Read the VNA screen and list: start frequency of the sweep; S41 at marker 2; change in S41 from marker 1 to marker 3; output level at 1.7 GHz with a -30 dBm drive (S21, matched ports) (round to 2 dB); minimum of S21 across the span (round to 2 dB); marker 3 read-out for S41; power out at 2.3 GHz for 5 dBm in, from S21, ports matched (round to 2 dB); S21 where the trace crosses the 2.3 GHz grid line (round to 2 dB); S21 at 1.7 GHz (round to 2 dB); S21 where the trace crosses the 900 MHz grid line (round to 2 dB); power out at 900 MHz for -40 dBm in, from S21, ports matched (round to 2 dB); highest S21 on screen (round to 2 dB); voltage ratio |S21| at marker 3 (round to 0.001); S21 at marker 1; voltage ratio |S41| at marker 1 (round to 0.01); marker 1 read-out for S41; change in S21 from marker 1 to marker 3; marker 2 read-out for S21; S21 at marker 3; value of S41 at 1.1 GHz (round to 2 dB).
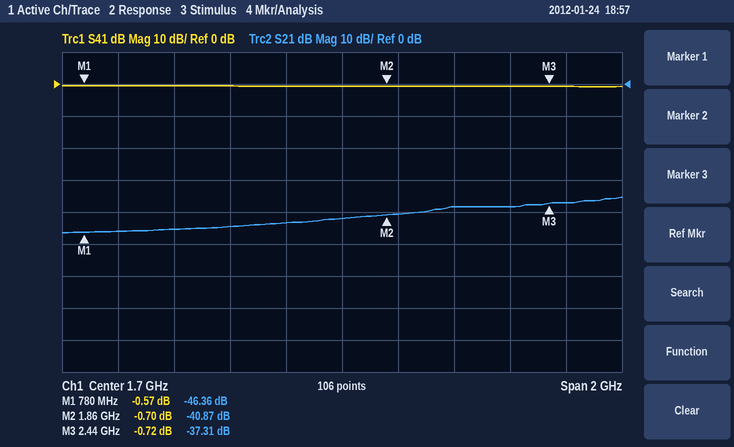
700 MHz
-0.70 dB
-0.15 dB
-72 dBm
-46 dB
-0.72 dB
-34 dBm
-38 dB
-42 dB
-46 dB
-86 dBm
-36 dB
0.014
-46.36 dB
0.94
-0.57 dB
9.05 dB
-40.87 dB
-37.31 dB
0 dB
